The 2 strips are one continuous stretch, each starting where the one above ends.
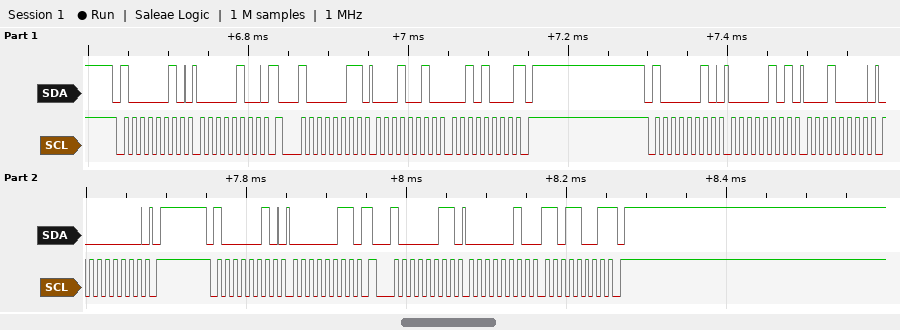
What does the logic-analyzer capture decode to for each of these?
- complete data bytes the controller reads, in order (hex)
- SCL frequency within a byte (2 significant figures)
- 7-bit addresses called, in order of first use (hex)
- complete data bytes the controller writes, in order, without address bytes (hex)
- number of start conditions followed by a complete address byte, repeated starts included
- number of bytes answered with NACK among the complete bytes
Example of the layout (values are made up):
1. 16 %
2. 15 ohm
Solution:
1. 12 28 02 D9
2. 100 kHz
3. 0x41
4. 04 05 10 00 03
5. 5
6. 2
